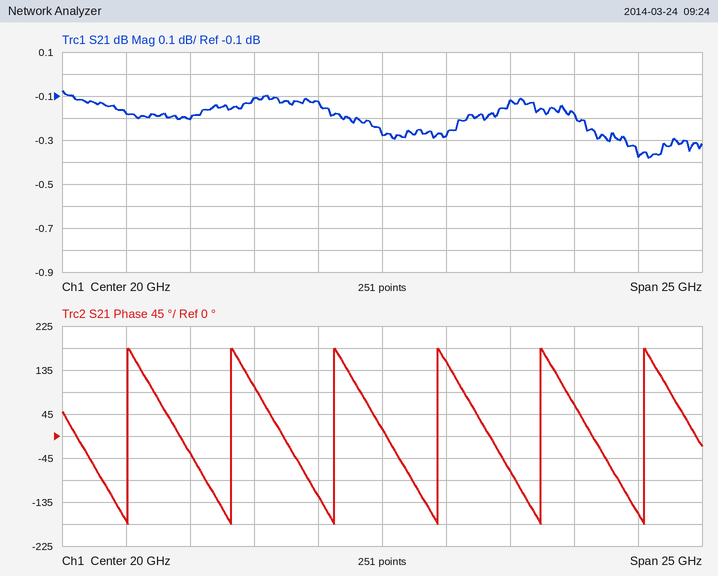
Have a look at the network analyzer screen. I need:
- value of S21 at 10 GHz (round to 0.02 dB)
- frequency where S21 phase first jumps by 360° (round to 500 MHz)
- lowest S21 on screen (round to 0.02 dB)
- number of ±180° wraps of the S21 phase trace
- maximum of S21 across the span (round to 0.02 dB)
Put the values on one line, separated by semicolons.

-0.18 dB; 10.0 GHz; -0.38 dB; 6; -0.08 dB
